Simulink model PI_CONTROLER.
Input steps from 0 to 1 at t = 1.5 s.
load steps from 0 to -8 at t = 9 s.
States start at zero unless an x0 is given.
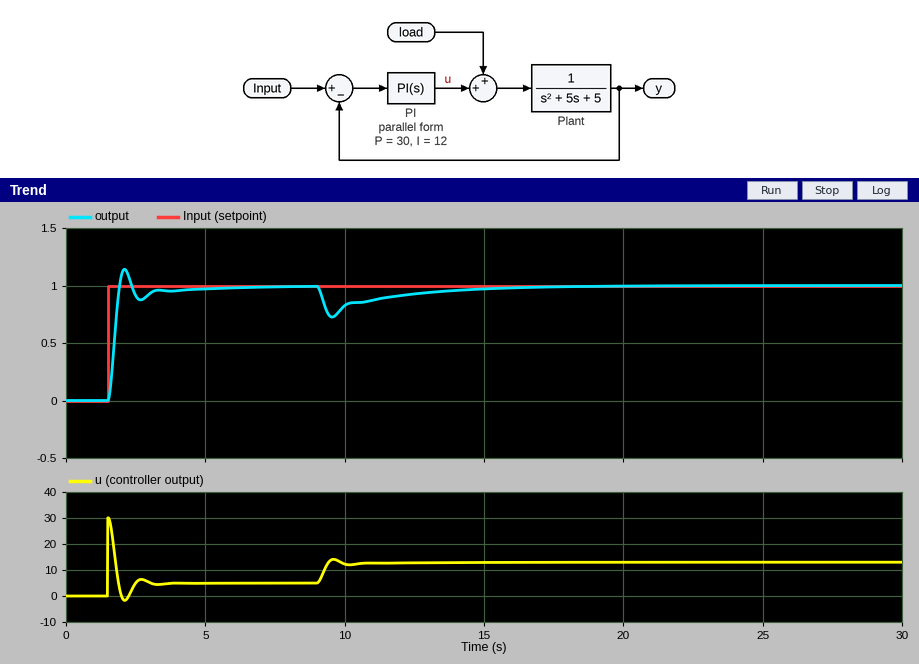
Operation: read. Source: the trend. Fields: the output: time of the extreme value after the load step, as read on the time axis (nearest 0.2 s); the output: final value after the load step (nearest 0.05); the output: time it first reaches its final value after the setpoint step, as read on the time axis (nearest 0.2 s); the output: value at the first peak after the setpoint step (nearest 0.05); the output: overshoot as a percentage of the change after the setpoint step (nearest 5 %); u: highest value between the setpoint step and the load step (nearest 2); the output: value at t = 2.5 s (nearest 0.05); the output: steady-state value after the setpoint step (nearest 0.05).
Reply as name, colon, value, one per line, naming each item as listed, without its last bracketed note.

the output: time of the extreme value after the load step, as read on the time axis: 9.6 s
the output: final value after the load step: 1.00
the output: time it first reaches its final value after the setpoint step, as read on the time axis: 2.0 s
the output: value at the first peak after the setpoint step: 1.15
the output: overshoot as a percentage of the change after the setpoint step: 15 %
u: highest value between the setpoint step and the load step: 30
the output: value at t = 2.5 s: 0.90
the output: steady-state value after the setpoint step: 1.00
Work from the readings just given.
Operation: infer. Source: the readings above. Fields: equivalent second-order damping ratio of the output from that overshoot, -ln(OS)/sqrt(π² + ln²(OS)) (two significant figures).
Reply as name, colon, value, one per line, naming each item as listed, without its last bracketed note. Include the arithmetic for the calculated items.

equivalent second-order damping ratio of the output from that overshoot, -ln(OS)/sqrt(π² + ln²(OS)): ln(0.15) = -1.897; 1.897 / sqrt(9.870 + 3.599) = 0.52
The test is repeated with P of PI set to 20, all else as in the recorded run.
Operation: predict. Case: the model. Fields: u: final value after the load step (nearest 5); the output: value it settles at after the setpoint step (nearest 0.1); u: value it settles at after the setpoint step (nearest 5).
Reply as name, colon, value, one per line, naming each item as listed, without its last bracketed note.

u: final value after the load step: 15
the output: value it settles at after the setpoint step: 1.0
u: value it settles at after the setpoint step: 5
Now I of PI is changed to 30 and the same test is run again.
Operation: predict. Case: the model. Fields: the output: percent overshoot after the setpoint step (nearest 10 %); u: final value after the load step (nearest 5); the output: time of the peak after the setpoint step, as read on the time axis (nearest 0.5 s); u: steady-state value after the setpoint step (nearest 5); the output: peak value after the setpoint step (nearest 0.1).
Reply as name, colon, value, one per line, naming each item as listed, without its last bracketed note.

the output: percent overshoot after the setpoint step: 30 %
u: final value after the load step: 15
the output: time of the peak after the setpoint step, as read on the time axis: 2.0 s
u: steady-state value after the setpoint step: 5
the output: peak value after the setpoint step: 1.3
